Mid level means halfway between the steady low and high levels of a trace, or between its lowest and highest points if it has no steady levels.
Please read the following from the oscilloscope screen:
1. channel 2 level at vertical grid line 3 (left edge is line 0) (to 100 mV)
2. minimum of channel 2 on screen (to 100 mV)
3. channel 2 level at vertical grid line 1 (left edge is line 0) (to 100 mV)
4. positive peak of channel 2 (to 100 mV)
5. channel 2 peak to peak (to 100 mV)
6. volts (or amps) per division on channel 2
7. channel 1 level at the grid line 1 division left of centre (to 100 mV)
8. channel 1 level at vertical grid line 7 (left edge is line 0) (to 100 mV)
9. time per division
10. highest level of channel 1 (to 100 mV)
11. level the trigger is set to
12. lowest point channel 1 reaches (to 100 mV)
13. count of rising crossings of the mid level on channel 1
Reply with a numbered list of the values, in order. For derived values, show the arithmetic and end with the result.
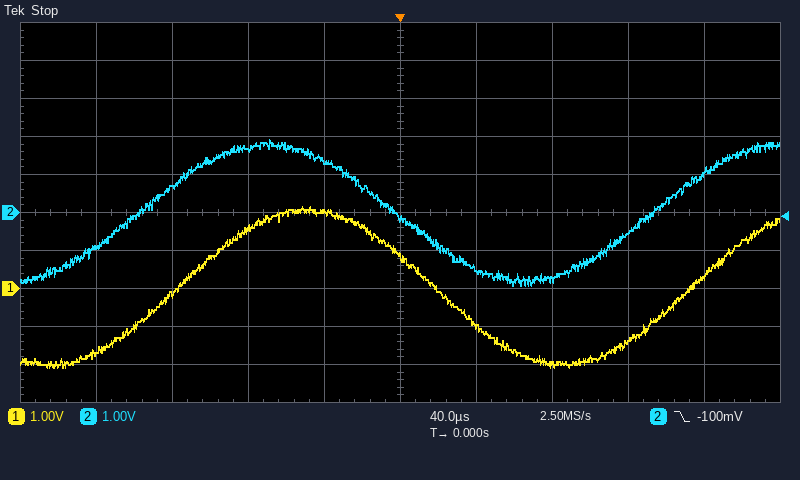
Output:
1. 1.7 V
2. -1.9 V
3. -900 mV
4. 1.9 V
5. 1.9 V − (-1.9 V) = 3.8 V
6. 1 V
7. 2.0 V
8. -2.0 V
9. 40 µs
10. 2.2 V
11. -100 mV
12. -2.1 V
13. 2
